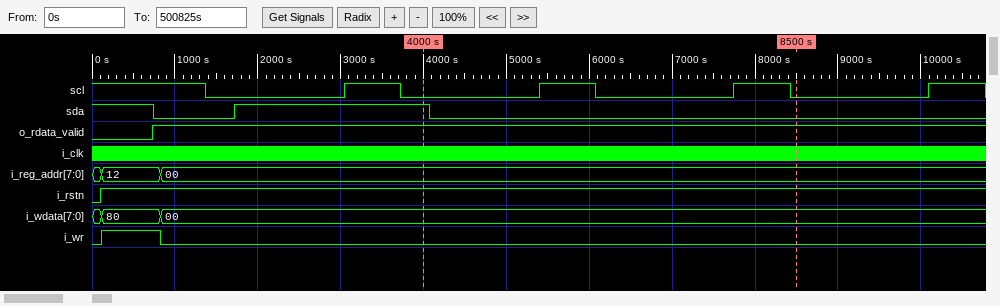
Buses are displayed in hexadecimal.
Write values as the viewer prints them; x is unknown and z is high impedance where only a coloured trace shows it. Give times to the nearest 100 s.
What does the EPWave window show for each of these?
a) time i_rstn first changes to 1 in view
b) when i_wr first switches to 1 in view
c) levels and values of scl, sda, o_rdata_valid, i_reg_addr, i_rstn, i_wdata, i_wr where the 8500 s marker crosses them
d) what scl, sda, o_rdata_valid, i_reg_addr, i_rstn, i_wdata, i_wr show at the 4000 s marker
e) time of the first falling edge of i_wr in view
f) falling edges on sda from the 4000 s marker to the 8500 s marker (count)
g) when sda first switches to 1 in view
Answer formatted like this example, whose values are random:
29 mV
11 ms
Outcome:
100 s
100 s
scl=0, sda=0, o_rdata_valid=1, i_reg_addr=00, i_rstn=1, i_wdata=00, i_wr=0
scl=0, sda=1, o_rdata_valid=1, i_reg_addr=00, i_rstn=1, i_wdata=00, i_wr=0
800 s
1
1700 s
